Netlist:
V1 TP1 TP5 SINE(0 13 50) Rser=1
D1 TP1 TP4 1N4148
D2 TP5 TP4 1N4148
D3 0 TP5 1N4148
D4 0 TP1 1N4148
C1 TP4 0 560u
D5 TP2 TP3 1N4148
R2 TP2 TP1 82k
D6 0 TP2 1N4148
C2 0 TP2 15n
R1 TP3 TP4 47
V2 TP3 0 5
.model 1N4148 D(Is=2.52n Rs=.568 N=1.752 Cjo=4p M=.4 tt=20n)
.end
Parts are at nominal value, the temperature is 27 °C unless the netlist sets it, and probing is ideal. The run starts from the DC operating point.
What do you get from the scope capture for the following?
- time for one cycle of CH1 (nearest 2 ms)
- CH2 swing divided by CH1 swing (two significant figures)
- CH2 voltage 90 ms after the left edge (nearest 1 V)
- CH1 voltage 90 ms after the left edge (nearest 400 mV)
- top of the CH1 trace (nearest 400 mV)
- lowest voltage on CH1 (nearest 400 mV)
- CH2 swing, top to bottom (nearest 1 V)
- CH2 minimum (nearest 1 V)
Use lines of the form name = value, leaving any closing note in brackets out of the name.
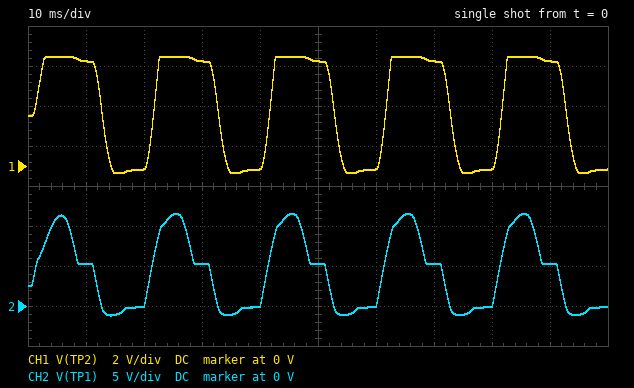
time for one cycle of CH1 = 20 ms
CH2 swing divided by CH1 swing = 2.2
CH2 voltage 90 ms after the left edge = 5 V
CH1 voltage 90 ms after the left edge = 5.2 V
top of the CH1 trace = 5.6 V
lowest voltage on CH1 = -400 mV
CH2 swing, top to bottom = 13 V
CH2 minimum = -1 V
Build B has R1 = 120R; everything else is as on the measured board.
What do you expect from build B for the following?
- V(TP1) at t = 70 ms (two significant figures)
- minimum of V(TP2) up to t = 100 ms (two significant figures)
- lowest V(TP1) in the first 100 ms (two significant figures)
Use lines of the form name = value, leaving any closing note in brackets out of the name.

V(TP1) at t = 70 ms = 5.2 V
minimum of V(TP2) up to t = 100 ms = -360 mV
lowest V(TP1) in the first 100 ms = -1.1 V
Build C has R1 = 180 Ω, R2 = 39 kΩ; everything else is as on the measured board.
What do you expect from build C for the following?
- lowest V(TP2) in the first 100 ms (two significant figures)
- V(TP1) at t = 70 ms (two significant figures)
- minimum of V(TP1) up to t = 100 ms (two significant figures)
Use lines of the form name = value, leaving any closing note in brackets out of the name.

lowest V(TP2) in the first 100 ms = -400 mV
V(TP1) at t = 70 ms = 5.2 V
minimum of V(TP1) up to t = 100 ms = -1.0 V
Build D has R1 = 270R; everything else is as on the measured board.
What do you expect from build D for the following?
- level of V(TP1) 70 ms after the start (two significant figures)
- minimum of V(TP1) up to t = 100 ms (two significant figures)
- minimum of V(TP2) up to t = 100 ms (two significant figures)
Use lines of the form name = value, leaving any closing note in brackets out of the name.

level of V(TP1) 70 ms after the start = 5.2 V
minimum of V(TP1) up to t = 100 ms = -1.0 V
minimum of V(TP2) up to t = 100 ms = -350 mV
